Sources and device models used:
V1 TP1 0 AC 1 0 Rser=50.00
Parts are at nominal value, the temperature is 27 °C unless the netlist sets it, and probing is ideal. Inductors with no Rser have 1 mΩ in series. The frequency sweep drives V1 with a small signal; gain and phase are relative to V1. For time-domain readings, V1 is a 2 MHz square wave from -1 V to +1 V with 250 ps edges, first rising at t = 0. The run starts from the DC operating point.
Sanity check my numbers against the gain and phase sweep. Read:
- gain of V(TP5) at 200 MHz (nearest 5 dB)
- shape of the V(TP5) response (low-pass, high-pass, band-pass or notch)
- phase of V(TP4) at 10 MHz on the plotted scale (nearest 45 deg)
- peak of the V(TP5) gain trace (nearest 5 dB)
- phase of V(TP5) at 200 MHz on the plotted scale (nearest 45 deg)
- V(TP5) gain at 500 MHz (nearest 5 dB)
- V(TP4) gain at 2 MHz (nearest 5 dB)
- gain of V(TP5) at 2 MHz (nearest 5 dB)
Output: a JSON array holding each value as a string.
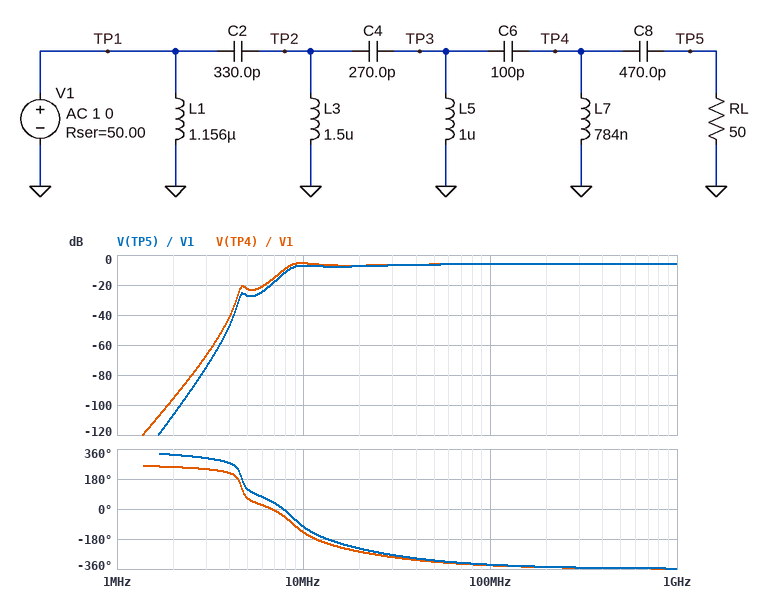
["-5 dB", "high-pass", "-135 deg", "-5 dB", "-360 deg", "-5 dB", "-95 dB", "-105 dB"]
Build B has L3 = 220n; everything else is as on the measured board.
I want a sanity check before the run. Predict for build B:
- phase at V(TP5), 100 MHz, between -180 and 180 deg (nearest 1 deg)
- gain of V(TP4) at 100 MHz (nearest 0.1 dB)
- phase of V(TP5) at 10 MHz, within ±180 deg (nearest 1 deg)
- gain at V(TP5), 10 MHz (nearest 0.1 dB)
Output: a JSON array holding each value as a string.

["35 deg", "-6.0 dB", "-60 deg", "-15.1 dB"]
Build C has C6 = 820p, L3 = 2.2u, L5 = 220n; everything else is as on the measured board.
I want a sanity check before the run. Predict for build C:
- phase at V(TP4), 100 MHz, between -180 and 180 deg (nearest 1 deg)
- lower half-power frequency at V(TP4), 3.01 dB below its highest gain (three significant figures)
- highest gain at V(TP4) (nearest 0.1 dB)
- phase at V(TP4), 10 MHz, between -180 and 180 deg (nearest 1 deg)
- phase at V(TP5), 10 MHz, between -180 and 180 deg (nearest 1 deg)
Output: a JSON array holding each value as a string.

["22 deg", "16.4 MHz", "-6.0 dB", "-162 deg", "-128 deg"]
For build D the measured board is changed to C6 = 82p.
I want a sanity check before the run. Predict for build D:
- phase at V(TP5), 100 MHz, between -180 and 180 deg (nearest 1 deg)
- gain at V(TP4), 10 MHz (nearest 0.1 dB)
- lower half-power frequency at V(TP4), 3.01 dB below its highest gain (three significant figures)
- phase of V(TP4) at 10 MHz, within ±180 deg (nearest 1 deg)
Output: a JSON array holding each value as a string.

["28 deg", "-6.5 dB", "8.60 MHz", "-129 deg"]
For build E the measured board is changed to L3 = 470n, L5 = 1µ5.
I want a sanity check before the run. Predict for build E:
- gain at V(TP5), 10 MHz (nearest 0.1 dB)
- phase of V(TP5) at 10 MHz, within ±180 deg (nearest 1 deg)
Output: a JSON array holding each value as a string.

["-11.6 dB", "-90 deg"]
